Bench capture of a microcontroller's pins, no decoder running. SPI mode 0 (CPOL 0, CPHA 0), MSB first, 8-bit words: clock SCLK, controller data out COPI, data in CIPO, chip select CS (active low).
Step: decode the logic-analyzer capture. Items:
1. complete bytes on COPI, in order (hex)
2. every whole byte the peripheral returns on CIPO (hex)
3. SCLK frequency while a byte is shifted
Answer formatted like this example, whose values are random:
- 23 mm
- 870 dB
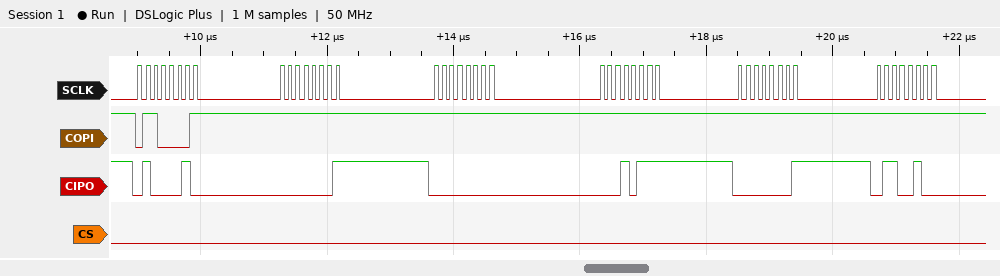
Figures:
- 61 FF FF FF FF FF
- 42 01 00 17 01 64
- 8 MHz
